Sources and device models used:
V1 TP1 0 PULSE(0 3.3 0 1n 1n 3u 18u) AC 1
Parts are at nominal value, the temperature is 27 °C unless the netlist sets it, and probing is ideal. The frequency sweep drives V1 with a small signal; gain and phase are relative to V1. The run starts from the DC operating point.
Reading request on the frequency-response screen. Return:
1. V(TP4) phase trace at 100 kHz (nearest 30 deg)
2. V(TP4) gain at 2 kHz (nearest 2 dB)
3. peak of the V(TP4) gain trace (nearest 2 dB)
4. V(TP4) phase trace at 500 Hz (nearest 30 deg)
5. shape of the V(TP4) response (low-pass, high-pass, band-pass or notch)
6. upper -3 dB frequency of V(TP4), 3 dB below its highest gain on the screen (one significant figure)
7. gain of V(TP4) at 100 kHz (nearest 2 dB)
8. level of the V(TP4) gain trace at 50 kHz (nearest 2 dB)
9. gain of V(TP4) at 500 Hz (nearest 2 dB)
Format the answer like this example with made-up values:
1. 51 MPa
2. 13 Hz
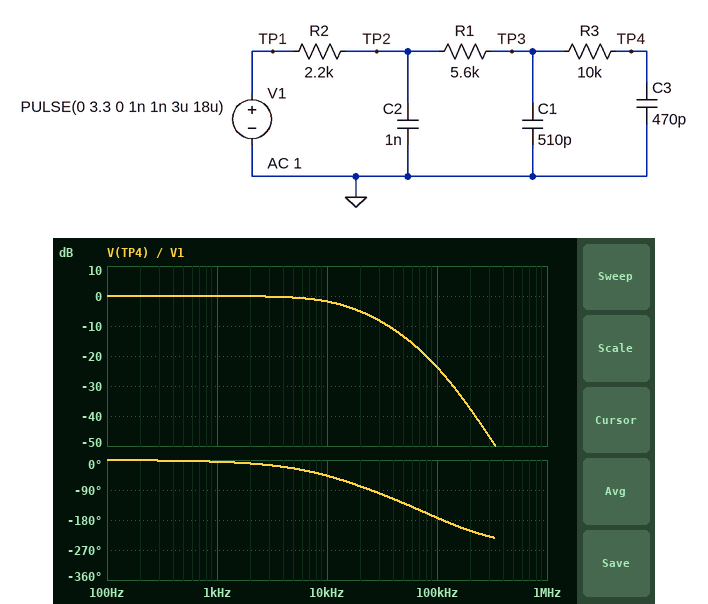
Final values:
1. -180 deg
2. 0 dB
3. 0 dB
4. 0 deg
5. low-pass
6. 10 kHz
7. -24 dB
8. -14 dB
9. 0 dB
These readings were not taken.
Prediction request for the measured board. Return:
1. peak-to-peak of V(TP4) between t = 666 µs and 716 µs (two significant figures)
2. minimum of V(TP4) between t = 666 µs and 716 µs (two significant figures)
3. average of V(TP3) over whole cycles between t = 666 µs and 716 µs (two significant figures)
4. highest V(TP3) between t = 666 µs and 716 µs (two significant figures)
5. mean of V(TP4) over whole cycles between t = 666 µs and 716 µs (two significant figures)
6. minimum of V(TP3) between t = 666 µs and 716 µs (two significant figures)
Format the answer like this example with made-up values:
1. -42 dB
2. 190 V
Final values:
1. 410 mV
2. 340 mV
3. 550 mV
4. 1.1 V
5. 550 mV
6. 210 mV
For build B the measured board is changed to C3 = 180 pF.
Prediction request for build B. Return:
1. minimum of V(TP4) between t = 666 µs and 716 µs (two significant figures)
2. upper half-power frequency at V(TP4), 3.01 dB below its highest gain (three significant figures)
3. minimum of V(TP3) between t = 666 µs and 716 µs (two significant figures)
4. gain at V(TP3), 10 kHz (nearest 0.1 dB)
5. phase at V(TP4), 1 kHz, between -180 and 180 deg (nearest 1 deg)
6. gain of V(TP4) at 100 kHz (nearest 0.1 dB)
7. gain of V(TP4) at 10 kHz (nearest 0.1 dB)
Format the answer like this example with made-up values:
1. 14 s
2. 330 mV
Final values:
1. 200 mV
2. 22.0 kHz
3. 160 mV
4. -0.7 dB
5. -3 deg
6. -17.4 dB
7. -0.8 dB
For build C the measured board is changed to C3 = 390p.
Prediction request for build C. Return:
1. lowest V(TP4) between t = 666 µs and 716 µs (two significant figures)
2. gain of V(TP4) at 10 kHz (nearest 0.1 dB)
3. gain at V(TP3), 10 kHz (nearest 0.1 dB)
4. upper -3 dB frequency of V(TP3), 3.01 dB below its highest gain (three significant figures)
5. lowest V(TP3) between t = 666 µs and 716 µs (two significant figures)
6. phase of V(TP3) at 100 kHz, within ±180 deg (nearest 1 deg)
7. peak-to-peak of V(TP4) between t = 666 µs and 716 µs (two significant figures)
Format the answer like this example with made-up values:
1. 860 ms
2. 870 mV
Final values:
1. 310 mV
2. -1.5 dB
3. -1.2 dB
4. 17.9 kHz
5. 200 mV
6. -103 deg
7. 470 mV
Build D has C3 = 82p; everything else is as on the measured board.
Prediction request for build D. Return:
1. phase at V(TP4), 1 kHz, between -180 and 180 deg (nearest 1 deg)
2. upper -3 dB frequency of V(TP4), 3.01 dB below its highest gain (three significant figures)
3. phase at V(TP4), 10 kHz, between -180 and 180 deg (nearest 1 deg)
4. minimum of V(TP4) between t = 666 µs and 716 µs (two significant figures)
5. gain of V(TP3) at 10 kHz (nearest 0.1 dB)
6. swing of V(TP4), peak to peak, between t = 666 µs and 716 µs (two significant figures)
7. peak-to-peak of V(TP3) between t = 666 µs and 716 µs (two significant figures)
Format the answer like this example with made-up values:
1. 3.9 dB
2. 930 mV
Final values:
1. -3 deg
2. 26.6 kHz
3. -27 deg
4. 140 mV
5. -0.5 dB
6. 950 mV
7. 1.0 V
